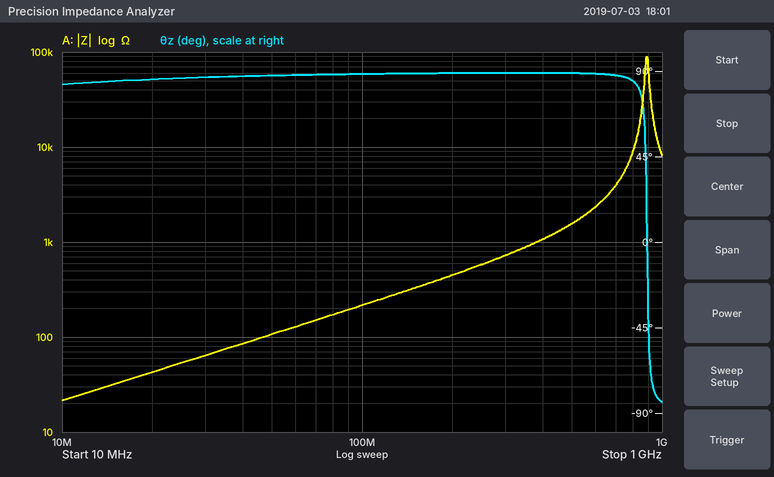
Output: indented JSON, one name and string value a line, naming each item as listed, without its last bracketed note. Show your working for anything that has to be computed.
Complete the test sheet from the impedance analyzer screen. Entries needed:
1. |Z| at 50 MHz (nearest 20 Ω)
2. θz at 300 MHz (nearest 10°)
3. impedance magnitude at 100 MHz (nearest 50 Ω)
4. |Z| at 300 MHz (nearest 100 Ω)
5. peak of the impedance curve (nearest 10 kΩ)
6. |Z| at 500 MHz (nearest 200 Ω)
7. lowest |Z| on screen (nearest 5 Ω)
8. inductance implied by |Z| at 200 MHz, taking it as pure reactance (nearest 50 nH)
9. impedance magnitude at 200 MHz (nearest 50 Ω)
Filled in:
{
  "|Z| at 50 MHz": "100 Ω",
  "θz at 300 MHz": "90°",
  "impedance magnitude at 100 MHz": "200 Ω",
  "|Z| at 300 MHz": "700 Ω",
  "peak of the impedance curve": "90 kΩ",
  "|Z| at 500 MHz": "1.6 kΩ",
  "lowest |Z| on screen": "20 Ω",
  "inductance implied by |Z| at 200 MHz, taking it as pure reactance": "L = 450 Ω/(2π × 200 MHz) ≈ 358 nH, so 350 nH to the nearest 50 nH",
  "impedance magnitude at 200 MHz": "450 Ω"
}
